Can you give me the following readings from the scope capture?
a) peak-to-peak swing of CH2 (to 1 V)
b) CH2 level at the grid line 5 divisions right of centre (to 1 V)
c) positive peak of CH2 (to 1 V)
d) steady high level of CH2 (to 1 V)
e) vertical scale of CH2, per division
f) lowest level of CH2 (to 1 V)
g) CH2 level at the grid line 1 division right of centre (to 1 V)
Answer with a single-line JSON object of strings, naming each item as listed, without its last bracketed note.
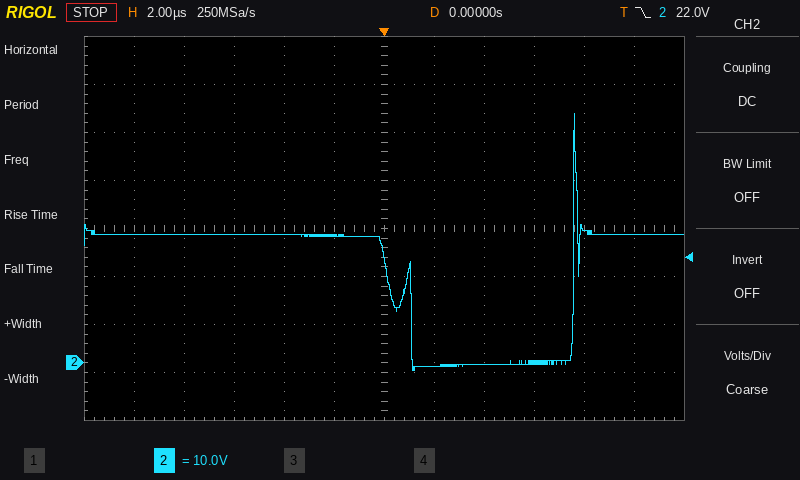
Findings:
{"peak-to-peak swing of CH2": "54 V", "CH2 level at the grid line 5 divisions right of centre": "27 V", "positive peak of CH2": "52 V", "steady high level of CH2": "27 V", "vertical scale of CH2, per division": "10 V", "lowest level of CH2": "-2 V", "CH2 level at the grid line 1 division right of centre": "-1 V"}
